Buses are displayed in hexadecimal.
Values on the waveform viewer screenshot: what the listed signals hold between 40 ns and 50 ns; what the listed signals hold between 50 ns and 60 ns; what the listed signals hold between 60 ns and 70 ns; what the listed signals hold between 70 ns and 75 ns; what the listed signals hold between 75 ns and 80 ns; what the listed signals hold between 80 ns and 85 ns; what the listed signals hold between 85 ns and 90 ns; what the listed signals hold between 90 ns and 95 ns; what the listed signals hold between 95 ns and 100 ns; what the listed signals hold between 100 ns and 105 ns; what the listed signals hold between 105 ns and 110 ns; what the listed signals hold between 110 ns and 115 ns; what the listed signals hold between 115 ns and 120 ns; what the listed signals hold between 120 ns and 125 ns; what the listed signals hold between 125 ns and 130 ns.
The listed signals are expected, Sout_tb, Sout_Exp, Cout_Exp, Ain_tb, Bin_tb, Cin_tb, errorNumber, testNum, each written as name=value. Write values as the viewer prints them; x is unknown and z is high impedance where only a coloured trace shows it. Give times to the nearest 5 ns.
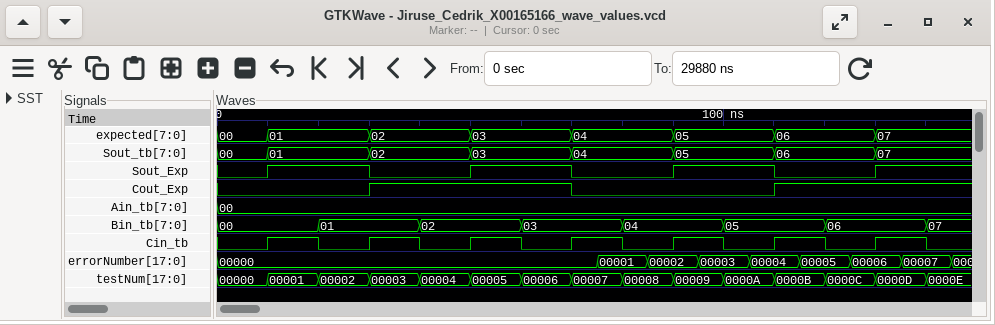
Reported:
expected=02, Sout_tb=02, Sout_Exp=0, Cout_Exp=1, Ain_tb=00, Bin_tb=02, Cin_tb=0, errorNumber=00000, testNum=00004
expected=03, Sout_tb=03, Sout_Exp=1, Cout_Exp=1, Ain_tb=00, Bin_tb=02, Cin_tb=1, errorNumber=00000, testNum=00005
expected=03, Sout_tb=03, Sout_Exp=1, Cout_Exp=1, Ain_tb=00, Bin_tb=03, Cin_tb=0, errorNumber=00000, testNum=00006
expected=04, Sout_tb=04, Sout_Exp=0, Cout_Exp=0, Ain_tb=00, Bin_tb=03, Cin_tb=1, errorNumber=00000, testNum=00007
expected=04, Sout_tb=04, Sout_Exp=0, Cout_Exp=0, Ain_tb=00, Bin_tb=03, Cin_tb=1, errorNumber=00001, testNum=00007
expected=04, Sout_tb=04, Sout_Exp=0, Cout_Exp=0, Ain_tb=00, Bin_tb=04, Cin_tb=0, errorNumber=00001, testNum=00008
expected=04, Sout_tb=04, Sout_Exp=0, Cout_Exp=0, Ain_tb=00, Bin_tb=04, Cin_tb=0, errorNumber=00002, testNum=00008
expected=05, Sout_tb=05, Sout_Exp=1, Cout_Exp=0, Ain_tb=00, Bin_tb=04, Cin_tb=1, errorNumber=00002, testNum=00009
expected=05, Sout_tb=05, Sout_Exp=1, Cout_Exp=0, Ain_tb=00, Bin_tb=04, Cin_tb=1, errorNumber=00003, testNum=00009
expected=05, Sout_tb=05, Sout_Exp=1, Cout_Exp=0, Ain_tb=00, Bin_tb=05, Cin_tb=0, errorNumber=00003, testNum=0000A
expected=05, Sout_tb=05, Sout_Exp=1, Cout_Exp=0, Ain_tb=00, Bin_tb=05, Cin_tb=0, errorNumber=00004, testNum=0000A
expected=06, Sout_tb=06, Sout_Exp=0, Cout_Exp=1, Ain_tb=00, Bin_tb=05, Cin_tb=1, errorNumber=00004, testNum=0000B
expected=06, Sout_tb=06, Sout_Exp=0, Cout_Exp=1, Ain_tb=00, Bin_tb=05, Cin_tb=1, errorNumber=00005, testNum=0000B
expected=06, Sout_tb=06, Sout_Exp=0, Cout_Exp=1, Ain_tb=00, Bin_tb=06, Cin_tb=0, errorNumber=00005, testNum=0000C
expected=06, Sout_tb=06, Sout_Exp=0, Cout_Exp=1, Ain_tb=00, Bin_tb=06, Cin_tb=0, errorNumber=00006, testNum=0000C
